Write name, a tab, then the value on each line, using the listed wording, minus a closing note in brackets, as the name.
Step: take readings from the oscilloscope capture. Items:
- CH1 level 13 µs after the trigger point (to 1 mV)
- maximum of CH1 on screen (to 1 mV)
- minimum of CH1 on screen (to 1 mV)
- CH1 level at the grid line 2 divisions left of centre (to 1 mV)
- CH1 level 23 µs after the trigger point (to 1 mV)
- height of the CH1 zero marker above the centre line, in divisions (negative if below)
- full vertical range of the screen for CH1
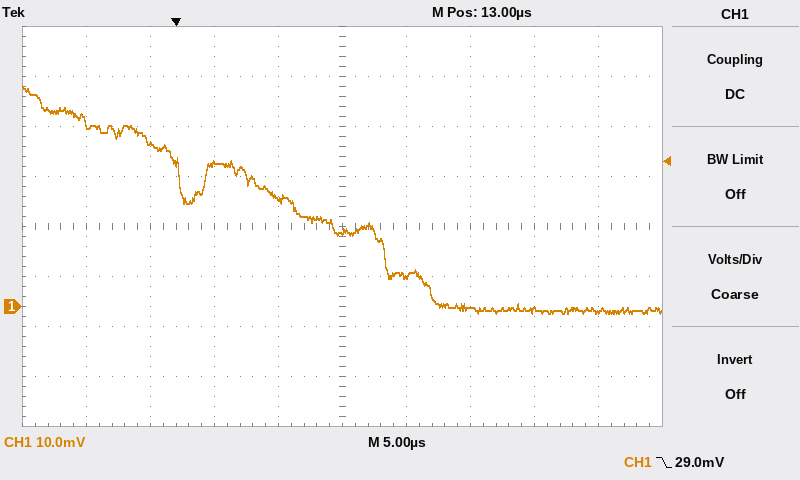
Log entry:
CH1 level 13 µs after the trigger point	15 mV
maximum of CH1 on screen	44 mV
minimum of CH1 on screen	-1 mV
CH1 level at the grid line 2 divisions left of centre	29 mV
CH1 level 23 µs after the trigger point	0 mV
height of the CH1 zero marker above the centre line, in divisions	-1.6 div
full vertical range of the screen for CH1	80 mV
